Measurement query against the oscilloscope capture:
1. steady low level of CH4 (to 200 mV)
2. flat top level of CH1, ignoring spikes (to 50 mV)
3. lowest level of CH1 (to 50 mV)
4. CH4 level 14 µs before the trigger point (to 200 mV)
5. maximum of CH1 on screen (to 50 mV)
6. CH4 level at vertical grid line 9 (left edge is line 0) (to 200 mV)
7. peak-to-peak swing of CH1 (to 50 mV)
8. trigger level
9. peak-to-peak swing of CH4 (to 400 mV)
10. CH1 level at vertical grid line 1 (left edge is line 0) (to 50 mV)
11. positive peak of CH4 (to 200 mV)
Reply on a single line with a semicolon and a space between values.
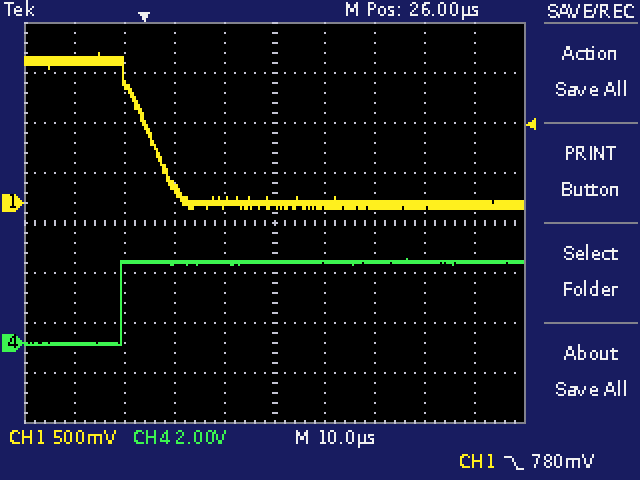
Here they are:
0.0 V; 1.40 V; -50 mV; 0.0 V; 1.50 V; 3.2 V; 1.55 V; 780 mV; 3.6 V; 1.40 V; 3.4 V
